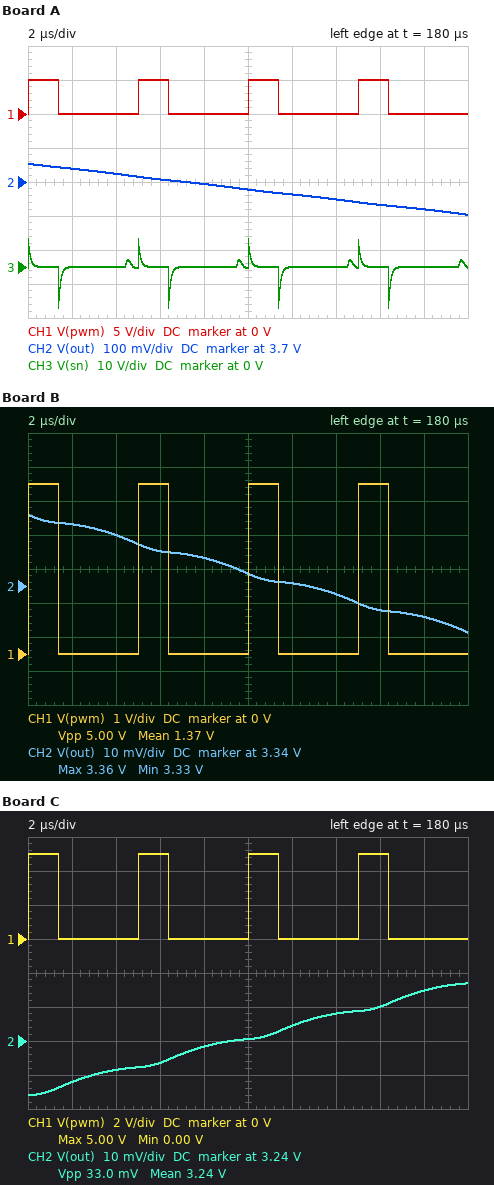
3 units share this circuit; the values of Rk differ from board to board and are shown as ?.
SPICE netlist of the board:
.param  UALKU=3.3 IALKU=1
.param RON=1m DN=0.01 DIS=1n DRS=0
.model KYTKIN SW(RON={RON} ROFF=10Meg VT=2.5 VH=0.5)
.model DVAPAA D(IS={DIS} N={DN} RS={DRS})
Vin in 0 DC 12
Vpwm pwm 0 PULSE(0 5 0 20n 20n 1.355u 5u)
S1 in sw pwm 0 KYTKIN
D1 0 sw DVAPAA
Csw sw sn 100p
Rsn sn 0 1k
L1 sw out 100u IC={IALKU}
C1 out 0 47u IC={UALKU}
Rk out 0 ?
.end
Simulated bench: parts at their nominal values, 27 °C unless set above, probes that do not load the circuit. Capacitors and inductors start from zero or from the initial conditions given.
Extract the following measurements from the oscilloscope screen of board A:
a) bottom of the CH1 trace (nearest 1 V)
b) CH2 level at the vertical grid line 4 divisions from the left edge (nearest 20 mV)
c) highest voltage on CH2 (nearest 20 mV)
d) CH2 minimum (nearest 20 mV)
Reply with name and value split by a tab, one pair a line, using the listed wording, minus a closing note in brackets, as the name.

bottom of the CH1 trace	0 V
CH2 level at the vertical grid line 4 divisions from the left edge	3.70 V
highest voltage on CH2	3.76 V
CH2 minimum	3.60 V
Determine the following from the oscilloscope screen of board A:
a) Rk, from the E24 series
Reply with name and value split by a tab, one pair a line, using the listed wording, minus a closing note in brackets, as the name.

Rk, from the E24 series	9.1 Ω
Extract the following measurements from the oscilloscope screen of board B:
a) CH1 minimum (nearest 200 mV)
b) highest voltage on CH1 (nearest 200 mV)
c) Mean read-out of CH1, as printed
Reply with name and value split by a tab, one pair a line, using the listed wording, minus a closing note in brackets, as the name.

CH1 minimum	0 V
highest voltage on CH1	5.0 V
Mean read-out of CH1, as printed	1.37 V
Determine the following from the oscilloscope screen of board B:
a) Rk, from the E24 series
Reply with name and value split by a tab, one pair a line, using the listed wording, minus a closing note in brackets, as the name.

Rk, from the E24 series	3.6 Ω
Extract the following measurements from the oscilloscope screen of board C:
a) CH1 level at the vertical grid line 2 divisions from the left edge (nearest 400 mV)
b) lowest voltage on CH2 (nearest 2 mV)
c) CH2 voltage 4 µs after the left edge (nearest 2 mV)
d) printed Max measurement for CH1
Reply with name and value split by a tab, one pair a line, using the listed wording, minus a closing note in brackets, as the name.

CH1 level at the vertical grid line 2 divisions from the left edge	0 V
lowest voltage on CH2	3.224 V
CH2 voltage 4 µs after the left edge	3.232 V
printed Max measurement for CH1	5.00 V
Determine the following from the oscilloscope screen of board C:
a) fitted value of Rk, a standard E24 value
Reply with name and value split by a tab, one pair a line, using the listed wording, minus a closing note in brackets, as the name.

fitted value of Rk, a standard E24 value	2.7 Ω
